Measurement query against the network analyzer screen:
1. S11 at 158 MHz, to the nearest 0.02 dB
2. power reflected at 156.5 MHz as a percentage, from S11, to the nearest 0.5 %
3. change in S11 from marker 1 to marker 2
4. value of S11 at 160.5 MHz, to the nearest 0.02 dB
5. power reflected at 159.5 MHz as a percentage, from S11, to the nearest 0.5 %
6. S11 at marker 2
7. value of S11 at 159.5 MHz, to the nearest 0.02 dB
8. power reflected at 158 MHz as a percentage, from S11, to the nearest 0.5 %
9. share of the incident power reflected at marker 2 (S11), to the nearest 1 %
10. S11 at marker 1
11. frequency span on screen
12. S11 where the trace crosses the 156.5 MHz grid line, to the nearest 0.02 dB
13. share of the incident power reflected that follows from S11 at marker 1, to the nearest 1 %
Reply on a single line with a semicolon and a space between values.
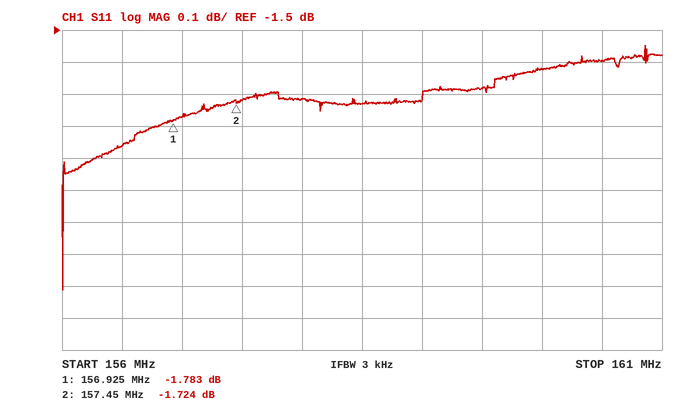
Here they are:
-1.72 dB; 65.0 %; 0.059 dB; -1.60 dB; 68.0 %; -1.724 dB; -1.68 dB; 67.5 %; 67 %; -1.783 dB; 5 MHz; -1.86 dB; 66 %
